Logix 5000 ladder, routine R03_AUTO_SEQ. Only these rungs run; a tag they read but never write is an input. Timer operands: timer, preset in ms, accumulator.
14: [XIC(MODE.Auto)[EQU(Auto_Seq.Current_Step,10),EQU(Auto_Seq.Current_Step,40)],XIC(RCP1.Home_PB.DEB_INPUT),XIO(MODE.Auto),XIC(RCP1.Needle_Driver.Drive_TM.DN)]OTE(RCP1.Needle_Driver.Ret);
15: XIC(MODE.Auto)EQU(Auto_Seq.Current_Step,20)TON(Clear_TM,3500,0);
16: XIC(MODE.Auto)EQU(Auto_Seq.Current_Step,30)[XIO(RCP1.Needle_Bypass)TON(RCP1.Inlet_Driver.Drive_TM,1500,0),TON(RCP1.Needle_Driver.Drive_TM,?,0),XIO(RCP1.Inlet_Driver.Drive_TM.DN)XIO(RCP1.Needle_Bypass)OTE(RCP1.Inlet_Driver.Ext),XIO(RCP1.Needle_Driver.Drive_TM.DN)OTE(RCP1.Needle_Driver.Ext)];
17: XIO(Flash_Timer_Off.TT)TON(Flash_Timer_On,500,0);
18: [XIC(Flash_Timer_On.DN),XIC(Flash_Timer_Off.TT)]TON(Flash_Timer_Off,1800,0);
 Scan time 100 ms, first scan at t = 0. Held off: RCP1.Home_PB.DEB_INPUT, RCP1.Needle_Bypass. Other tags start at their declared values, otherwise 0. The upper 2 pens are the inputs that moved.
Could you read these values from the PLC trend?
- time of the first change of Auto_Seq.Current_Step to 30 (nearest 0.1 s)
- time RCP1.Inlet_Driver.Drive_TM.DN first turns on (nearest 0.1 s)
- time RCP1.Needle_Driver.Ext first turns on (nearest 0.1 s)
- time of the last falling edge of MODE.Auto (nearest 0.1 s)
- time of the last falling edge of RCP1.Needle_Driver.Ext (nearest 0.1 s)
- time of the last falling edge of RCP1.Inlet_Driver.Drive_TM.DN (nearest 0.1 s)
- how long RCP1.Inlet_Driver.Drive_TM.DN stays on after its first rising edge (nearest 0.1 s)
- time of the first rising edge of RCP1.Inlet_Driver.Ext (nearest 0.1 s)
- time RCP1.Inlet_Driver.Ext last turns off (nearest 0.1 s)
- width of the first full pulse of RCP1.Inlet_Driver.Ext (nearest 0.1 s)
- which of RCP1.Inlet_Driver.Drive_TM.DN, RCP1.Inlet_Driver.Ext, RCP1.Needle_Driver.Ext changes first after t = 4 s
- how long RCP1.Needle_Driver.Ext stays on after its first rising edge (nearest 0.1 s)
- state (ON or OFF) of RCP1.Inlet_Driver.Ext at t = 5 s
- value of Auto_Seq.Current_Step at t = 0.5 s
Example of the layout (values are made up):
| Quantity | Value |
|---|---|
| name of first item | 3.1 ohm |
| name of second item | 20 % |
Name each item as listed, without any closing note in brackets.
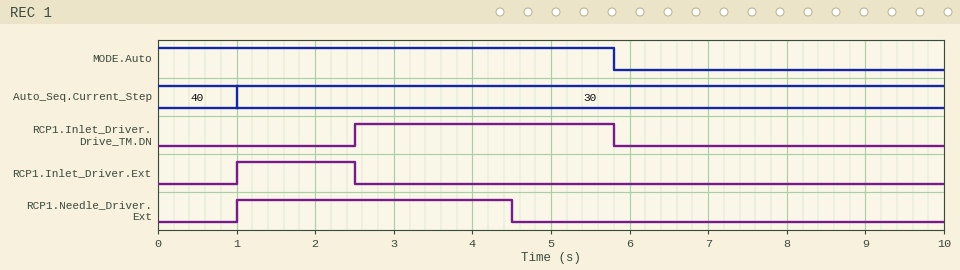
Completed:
| Quantity | Value |
|---|---|
| time of the first change of Auto_Seq.Current_Step to 30 | 1.0 s |
| time RCP1.Inlet_Driver.Drive_TM.DN first turns on | 2.5 s |
| time RCP1.Needle_Driver.Ext first turns on | 1.0 s |
| time of the last falling edge of MODE.Auto | 5.8 s |
| time of the last falling edge of RCP1.Needle_Driver.Ext | 4.5 s |
| time of the last falling edge of RCP1.Inlet_Driver.Drive_TM.DN | 5.8 s |
| how long RCP1.Inlet_Driver.Drive_TM.DN stays on after its first rising edge | 3.3 s |
| time of the first rising edge of RCP1.Inlet_Driver.Ext | 1.0 s |
| time RCP1.Inlet_Driver.Ext last turns off | 2.5 s |
| width of the first full pulse of RCP1.Inlet_Driver.Ext | 1.5 s |
| which of RCP1.Inlet_Driver.Drive_TM.DN, RCP1.Inlet_Driver.Ext, RCP1.Needle_Driver.Ext changes first after t = 4 s | RCP1.Needle_Driver.Ext |
| how long RCP1.Needle_Driver.Ext stays on after its first rising edge | 3.5 s |
| state (ON or OFF) of RCP1.Inlet_Driver.Ext at t = 5 s | OFF |
| value of Auto_Seq.Current_Step at t = 0.5 s | 40 |
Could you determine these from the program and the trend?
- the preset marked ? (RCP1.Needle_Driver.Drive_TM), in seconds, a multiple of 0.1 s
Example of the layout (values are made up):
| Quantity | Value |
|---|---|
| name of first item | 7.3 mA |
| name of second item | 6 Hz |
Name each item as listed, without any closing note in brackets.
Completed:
| Quantity | Value |
|---|---|
| the preset marked ? (RCP1.Needle_Driver.Drive_TM), in seconds, a multiple of 0.1 s | 3.5 s |
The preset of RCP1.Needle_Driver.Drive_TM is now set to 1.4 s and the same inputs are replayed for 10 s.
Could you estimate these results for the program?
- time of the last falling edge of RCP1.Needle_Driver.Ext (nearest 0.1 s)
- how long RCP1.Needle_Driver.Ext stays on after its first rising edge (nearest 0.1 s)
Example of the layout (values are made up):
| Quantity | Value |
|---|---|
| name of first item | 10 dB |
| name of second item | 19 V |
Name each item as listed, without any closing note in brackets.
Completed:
| Quantity | Value |
|---|---|
| time of the last falling edge of RCP1.Needle_Driver.Ext | 2.4 s |
| how long RCP1.Needle_Driver.Ext stays on after its first rising edge | 1.4 s |
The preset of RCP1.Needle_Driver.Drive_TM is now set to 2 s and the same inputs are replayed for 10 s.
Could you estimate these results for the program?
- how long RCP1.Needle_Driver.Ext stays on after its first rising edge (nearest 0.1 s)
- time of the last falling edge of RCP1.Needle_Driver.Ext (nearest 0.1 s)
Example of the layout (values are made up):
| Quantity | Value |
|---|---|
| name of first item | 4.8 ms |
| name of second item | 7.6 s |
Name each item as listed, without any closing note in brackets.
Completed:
| Quantity | Value |
|---|---|
| how long RCP1.Needle_Driver.Ext stays on after its first rising edge | 2.0 s |
| time of the last falling edge of RCP1.Needle_Driver.Ext | 3.0 s |
